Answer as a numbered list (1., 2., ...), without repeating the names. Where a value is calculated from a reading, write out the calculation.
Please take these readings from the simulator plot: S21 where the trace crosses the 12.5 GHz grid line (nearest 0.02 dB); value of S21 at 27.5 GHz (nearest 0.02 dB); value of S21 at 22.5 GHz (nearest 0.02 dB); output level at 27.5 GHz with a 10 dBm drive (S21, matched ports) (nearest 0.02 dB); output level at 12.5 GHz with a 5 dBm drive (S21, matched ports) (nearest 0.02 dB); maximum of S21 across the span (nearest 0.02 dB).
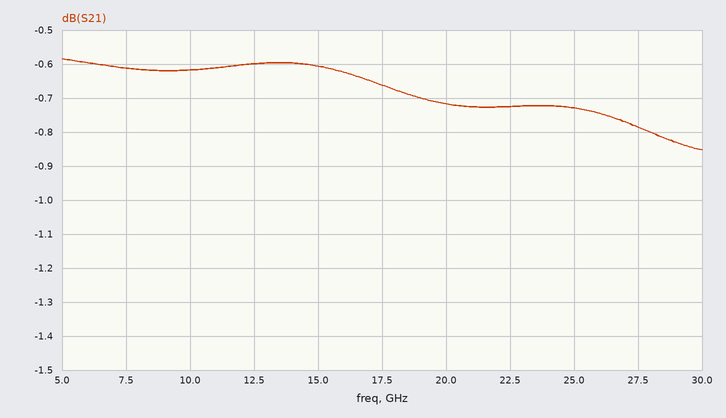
1. -0.60 dB
2. -0.78 dB
3. -0.72 dB
4. 10 dBm + (-0.78 dB) = 9.22 dBm
5. 5 dBm + (-0.60 dB) = 4.40 dBm
6. -0.58 dB
